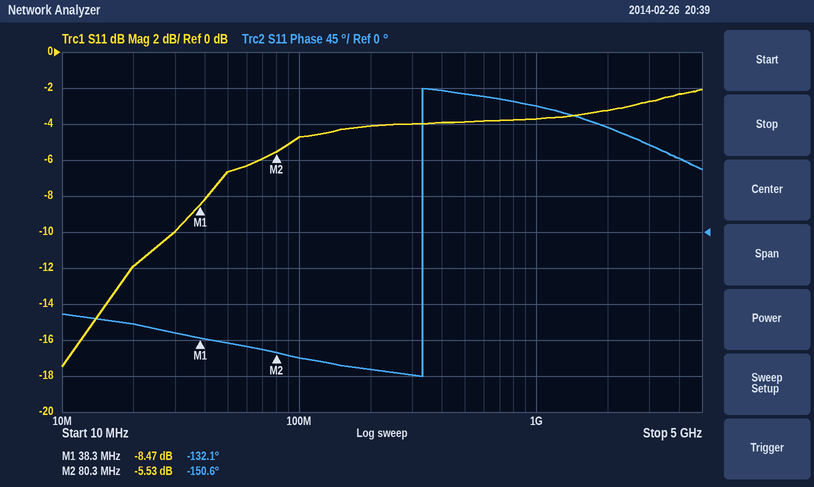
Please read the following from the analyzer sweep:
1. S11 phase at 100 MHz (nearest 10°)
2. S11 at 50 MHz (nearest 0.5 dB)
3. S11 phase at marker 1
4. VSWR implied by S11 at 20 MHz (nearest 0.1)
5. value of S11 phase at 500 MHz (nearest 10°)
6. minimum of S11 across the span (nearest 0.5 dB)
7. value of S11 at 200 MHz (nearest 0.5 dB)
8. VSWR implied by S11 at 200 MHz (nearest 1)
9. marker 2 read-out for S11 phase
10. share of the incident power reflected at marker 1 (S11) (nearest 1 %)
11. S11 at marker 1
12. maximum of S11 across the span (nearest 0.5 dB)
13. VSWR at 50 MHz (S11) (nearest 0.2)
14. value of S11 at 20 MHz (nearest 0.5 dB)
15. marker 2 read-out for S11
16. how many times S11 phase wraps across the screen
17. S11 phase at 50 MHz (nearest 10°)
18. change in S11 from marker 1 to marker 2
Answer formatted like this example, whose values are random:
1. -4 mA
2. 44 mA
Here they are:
1. -160°
2. -6.5 dB
3. -132.1°
4. 1.7
5. 170°
6. -17.5 dB
7. -4.0 dB
8. 4
9. -150.6°
10. 14 %
11. -8.47 dB
12. -2.0 dB
13. 2.8
14. -12.0 dB
15. -5.53 dB
16. 1
17. -140°
18. 2.94 dB
